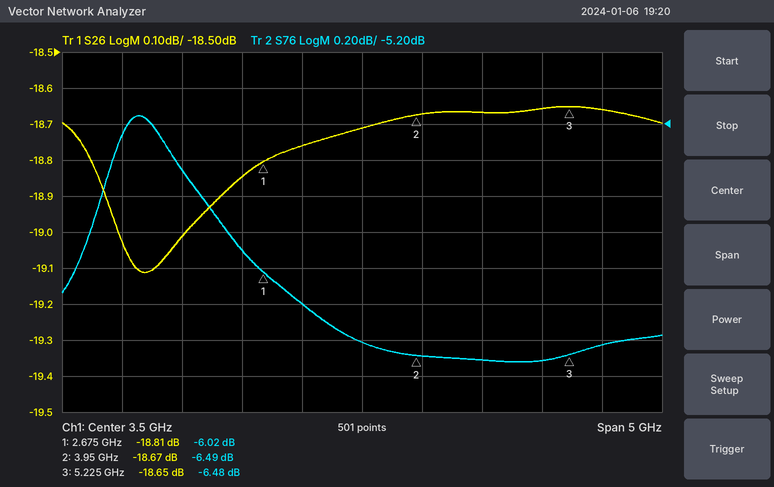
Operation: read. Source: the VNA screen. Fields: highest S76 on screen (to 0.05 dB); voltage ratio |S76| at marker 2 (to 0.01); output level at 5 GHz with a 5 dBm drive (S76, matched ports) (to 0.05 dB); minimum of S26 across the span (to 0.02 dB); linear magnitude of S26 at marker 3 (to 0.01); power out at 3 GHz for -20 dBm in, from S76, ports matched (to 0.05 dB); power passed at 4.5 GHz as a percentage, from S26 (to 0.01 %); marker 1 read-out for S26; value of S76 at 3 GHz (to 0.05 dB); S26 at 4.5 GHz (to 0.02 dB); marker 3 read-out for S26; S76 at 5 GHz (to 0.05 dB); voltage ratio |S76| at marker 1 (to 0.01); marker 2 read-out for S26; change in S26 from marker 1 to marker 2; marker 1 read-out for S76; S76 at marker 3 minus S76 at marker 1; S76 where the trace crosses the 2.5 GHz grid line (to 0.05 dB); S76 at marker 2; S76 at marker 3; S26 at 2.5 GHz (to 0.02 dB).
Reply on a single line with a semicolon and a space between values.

-5.15 dB; 0.47; -1.50 dBm; -19.12 dB; 0.12; -26.20 dBm; 1.36 %; -18.81 dB; -6.20 dB; -18.66 dB; -18.65 dB; -6.50 dB; 0.50; -18.67 dB; 0.14 dB; -6.02 dB; -0.46 dB; -5.90 dB; -6.49 dB; -6.48 dB; -18.84 dB
